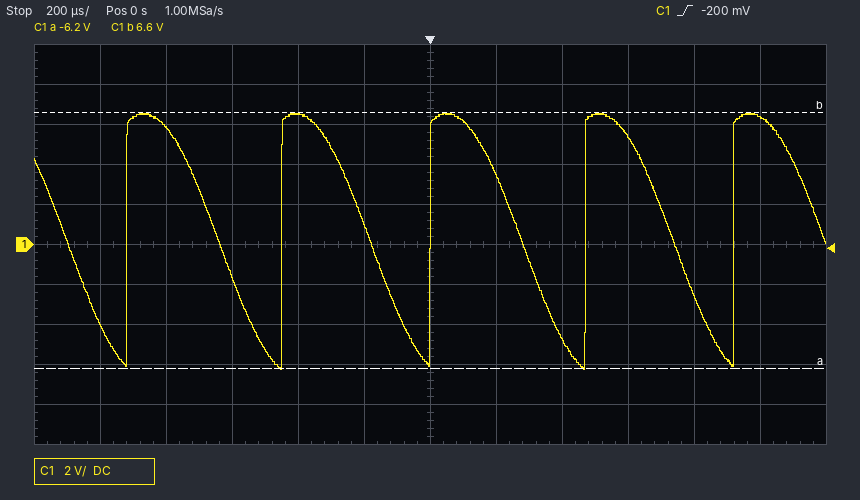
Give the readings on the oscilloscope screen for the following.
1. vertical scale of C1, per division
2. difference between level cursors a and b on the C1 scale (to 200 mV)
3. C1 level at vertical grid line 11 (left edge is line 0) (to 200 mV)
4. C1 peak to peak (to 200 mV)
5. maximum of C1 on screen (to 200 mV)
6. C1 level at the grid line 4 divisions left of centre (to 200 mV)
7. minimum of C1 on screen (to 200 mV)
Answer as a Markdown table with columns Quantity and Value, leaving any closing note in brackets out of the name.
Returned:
| Quantity | Value |
|---|---|
| vertical scale of C1, per division | 2 V |
| difference between level cursors a and b on the C1 scale | 12.8 V |
| C1 level at vertical grid line 11 (left edge is line 0) | 6.4 V |
| C1 peak to peak | 12.8 V |
| maximum of C1 on screen | 6.6 V |
| C1 level at the grid line 4 divisions left of centre | 5.8 V |
| minimum of C1 on screen | -6.2 V |
